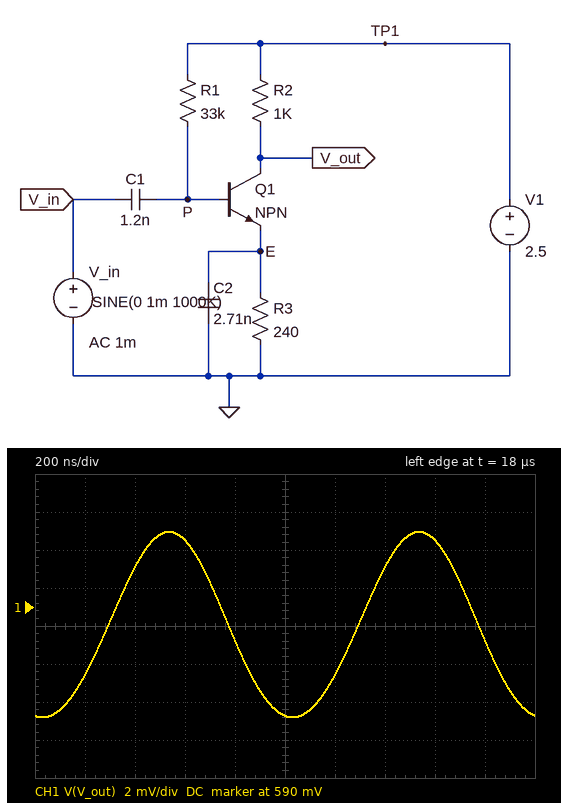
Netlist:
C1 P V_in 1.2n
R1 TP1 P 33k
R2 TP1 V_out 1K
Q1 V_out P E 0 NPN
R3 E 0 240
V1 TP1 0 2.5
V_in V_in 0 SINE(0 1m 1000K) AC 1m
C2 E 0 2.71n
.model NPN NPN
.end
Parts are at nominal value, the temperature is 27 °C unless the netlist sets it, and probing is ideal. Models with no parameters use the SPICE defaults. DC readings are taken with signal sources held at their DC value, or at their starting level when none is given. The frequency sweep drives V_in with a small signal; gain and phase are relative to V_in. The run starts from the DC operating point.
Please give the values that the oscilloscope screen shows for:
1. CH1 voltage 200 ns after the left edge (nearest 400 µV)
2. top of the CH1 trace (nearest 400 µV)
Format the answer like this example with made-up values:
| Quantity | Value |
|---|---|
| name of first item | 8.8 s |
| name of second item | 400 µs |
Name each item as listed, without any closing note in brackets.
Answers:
| Quantity | Value |
|---|---|
| CH1 voltage 200 ns after the left edge | 586.4 mV |
| top of the CH1 trace | 594.0 mV |
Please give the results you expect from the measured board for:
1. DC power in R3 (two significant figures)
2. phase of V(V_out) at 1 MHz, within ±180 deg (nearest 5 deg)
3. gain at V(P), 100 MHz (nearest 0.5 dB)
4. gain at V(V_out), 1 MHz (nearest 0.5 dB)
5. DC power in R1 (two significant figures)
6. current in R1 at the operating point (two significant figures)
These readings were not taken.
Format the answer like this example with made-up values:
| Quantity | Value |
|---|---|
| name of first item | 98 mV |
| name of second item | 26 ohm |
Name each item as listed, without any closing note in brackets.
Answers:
| Quantity | Value |
|---|---|
| DC power in R3 | 910 µW |
| phase of V(V_out) at 1 MHz, within ±180 deg | -100 deg |
| gain at V(P), 100 MHz | 0 dB |
| gain at V(V_out), 1 MHz | 13.5 dB |
| DC power in R1 | 47 µW |
| current in R1 at the operating point | 38 µA |
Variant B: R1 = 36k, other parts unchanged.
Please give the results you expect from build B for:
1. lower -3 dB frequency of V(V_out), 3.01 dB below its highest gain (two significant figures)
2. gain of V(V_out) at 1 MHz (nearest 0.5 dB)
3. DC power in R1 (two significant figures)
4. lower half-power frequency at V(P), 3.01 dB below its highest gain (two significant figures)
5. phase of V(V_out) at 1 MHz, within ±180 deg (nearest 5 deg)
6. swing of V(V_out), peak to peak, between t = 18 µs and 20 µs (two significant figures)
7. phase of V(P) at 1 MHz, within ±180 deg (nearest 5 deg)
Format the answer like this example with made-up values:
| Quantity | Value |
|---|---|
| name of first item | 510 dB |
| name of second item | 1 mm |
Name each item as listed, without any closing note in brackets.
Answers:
| Quantity | Value |
|---|---|
| lower -3 dB frequency of V(V_out), 3.01 dB below its highest gain | 6.2 MHz |
| gain of V(V_out) at 1 MHz | 15.0 dB |
| DC power in R1 | 43 µW |
| lower half-power frequency at V(P), 3.01 dB below its highest gain | 3.7 MHz |
| phase of V(V_out) at 1 MHz, within ±180 deg | -105 deg |
| swing of V(V_out), peak to peak, between t = 18 µs and 20 µs | 11 mV |
| phase of V(P) at 1 MHz, within ±180 deg | 15 deg |
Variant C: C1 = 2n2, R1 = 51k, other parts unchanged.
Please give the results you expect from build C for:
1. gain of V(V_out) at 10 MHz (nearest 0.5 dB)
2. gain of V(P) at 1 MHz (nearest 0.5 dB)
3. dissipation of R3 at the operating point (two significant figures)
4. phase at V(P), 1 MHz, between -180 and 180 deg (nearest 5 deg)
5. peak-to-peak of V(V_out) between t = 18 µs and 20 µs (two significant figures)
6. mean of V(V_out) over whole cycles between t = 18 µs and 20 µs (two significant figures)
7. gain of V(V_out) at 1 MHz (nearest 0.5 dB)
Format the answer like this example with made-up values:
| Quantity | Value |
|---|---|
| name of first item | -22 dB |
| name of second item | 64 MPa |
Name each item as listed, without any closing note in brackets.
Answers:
| Quantity | Value |
|---|---|
| gain of V(V_out) at 10 MHz | 33.5 dB |
| gain of V(P) at 1 MHz | -1.5 dB |
| dissipation of R3 at the operating point | 880 µW |
| phase at V(P), 1 MHz, between -180 and 180 deg | 5 deg |
| peak-to-peak of V(V_out) between t = 18 µs and 20 µs | 22 mV |
| mean of V(V_out) over whole cycles between t = 18 µs and 20 µs | 610 mV |
| gain of V(V_out) at 1 MHz | 20.5 dB |
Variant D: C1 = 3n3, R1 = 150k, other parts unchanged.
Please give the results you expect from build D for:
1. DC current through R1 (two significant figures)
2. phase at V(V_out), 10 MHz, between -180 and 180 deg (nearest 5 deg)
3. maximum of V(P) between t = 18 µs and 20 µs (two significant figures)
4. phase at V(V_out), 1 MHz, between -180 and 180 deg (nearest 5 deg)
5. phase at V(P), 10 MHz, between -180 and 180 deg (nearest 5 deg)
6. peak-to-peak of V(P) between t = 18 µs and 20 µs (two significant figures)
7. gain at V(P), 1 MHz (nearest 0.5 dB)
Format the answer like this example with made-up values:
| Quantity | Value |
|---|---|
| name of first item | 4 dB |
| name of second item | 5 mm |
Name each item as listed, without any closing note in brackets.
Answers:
| Quantity | Value |
|---|---|
| DC current through R1 | 9.9 µA |
| phase at V(V_out), 10 MHz, between -180 and 180 deg | -165 deg |
| maximum of V(P) between t = 18 µs and 20 µs | 1.0 V |
| phase at V(V_out), 1 MHz, between -180 and 180 deg | -125 deg |
| phase at V(P), 10 MHz, between -180 and 180 deg | 0 deg |
| peak-to-peak of V(P) between t = 18 µs and 20 µs | 2.0 mV |
| gain at V(P), 1 MHz | 0 dB |
